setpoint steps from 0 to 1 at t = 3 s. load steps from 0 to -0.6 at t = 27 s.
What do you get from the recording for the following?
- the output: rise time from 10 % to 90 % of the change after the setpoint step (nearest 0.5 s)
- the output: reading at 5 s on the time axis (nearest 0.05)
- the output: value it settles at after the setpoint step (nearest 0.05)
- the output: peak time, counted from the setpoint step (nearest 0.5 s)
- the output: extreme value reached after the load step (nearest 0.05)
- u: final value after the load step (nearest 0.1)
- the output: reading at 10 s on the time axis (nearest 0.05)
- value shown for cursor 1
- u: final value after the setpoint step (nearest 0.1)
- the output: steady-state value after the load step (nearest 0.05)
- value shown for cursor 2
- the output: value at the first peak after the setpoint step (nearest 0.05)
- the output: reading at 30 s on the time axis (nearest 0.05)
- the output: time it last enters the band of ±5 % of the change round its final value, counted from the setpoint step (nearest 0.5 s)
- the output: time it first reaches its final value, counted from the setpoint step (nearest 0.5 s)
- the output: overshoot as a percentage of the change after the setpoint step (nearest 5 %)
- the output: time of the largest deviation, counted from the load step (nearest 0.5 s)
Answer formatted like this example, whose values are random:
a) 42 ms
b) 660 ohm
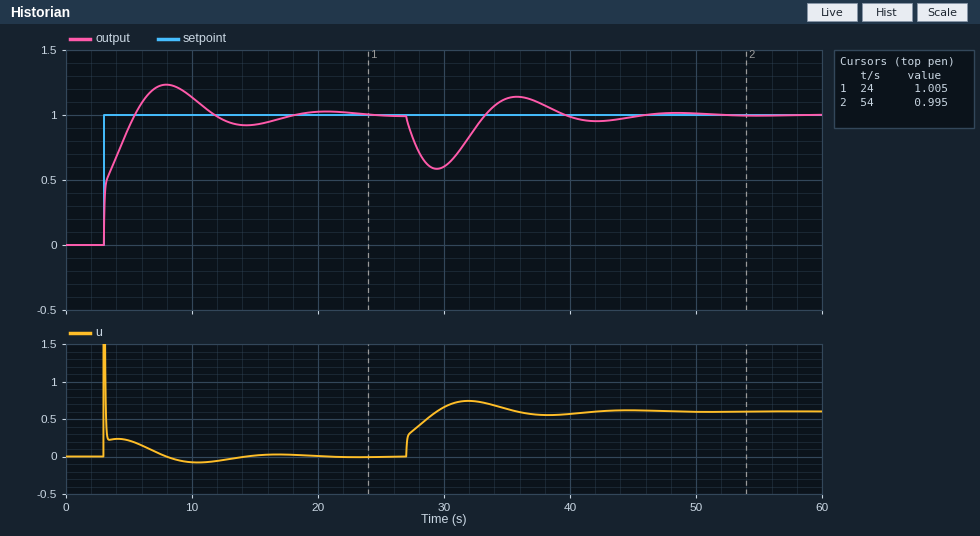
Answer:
a) 2.0 s
b) 0.90
c) 1.00
d) 5.0 s
e) 0.60
f) 0.6
g) 1.15
h) 1.005
i) 0.0
j) 1.00
k) 0.995
l) 1.25
m) 0.60
n) 13.0 s
o) 2.5 s
p) 25 %
q) 2.5 s
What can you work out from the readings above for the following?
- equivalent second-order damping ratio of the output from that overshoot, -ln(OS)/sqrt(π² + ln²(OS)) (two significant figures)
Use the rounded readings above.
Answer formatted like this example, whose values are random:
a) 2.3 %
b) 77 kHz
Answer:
a) 0.40
